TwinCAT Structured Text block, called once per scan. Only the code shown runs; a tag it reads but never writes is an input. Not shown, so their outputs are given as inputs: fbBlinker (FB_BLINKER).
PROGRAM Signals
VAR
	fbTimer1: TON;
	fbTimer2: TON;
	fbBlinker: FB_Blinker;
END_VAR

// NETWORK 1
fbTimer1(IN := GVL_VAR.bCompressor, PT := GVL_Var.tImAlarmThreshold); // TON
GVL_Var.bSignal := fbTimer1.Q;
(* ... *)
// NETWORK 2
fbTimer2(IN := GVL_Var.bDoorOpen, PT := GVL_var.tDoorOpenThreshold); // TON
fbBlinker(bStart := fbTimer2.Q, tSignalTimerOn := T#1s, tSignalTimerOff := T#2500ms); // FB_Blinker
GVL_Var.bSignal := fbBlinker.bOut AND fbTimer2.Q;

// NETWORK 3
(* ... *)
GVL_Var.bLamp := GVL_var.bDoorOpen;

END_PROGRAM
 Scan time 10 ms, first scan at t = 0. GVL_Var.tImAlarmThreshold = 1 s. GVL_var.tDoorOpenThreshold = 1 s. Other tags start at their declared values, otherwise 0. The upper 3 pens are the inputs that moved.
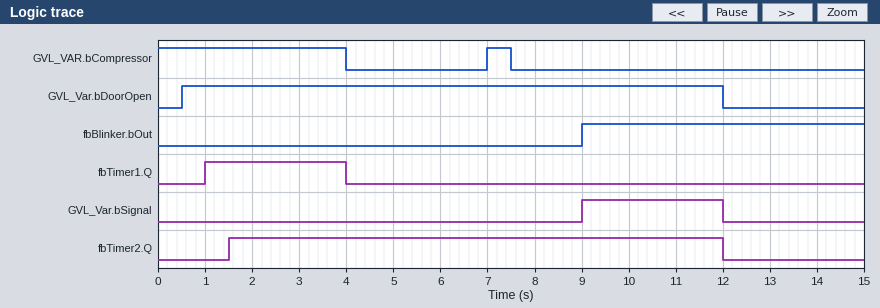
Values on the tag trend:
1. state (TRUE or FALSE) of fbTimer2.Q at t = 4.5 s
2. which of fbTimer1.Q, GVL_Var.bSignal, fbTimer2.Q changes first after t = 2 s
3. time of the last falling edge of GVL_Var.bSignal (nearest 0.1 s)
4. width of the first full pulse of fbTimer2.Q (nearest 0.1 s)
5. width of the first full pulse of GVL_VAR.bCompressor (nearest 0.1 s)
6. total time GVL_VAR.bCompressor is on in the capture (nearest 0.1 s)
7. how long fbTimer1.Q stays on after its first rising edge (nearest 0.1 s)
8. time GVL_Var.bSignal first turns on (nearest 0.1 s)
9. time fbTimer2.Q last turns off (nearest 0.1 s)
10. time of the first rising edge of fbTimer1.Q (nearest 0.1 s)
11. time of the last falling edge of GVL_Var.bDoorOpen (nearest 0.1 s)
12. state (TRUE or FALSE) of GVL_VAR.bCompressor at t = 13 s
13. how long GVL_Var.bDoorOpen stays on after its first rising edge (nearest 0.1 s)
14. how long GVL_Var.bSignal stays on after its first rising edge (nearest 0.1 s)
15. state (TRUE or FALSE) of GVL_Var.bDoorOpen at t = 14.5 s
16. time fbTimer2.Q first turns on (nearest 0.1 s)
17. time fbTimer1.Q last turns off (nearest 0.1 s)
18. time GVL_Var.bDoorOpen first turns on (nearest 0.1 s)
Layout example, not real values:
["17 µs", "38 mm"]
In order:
["TRUE", "fbTimer1.Q", "12.0 s", "10.5 s", "0.5 s", "4.5 s", "3.0 s", "9.0 s", "12.0 s", "1.0 s", "12.0 s", "FALSE", "11.5 s", "3.0 s", "FALSE", "1.5 s", "4.0 s", "0.5 s"]
